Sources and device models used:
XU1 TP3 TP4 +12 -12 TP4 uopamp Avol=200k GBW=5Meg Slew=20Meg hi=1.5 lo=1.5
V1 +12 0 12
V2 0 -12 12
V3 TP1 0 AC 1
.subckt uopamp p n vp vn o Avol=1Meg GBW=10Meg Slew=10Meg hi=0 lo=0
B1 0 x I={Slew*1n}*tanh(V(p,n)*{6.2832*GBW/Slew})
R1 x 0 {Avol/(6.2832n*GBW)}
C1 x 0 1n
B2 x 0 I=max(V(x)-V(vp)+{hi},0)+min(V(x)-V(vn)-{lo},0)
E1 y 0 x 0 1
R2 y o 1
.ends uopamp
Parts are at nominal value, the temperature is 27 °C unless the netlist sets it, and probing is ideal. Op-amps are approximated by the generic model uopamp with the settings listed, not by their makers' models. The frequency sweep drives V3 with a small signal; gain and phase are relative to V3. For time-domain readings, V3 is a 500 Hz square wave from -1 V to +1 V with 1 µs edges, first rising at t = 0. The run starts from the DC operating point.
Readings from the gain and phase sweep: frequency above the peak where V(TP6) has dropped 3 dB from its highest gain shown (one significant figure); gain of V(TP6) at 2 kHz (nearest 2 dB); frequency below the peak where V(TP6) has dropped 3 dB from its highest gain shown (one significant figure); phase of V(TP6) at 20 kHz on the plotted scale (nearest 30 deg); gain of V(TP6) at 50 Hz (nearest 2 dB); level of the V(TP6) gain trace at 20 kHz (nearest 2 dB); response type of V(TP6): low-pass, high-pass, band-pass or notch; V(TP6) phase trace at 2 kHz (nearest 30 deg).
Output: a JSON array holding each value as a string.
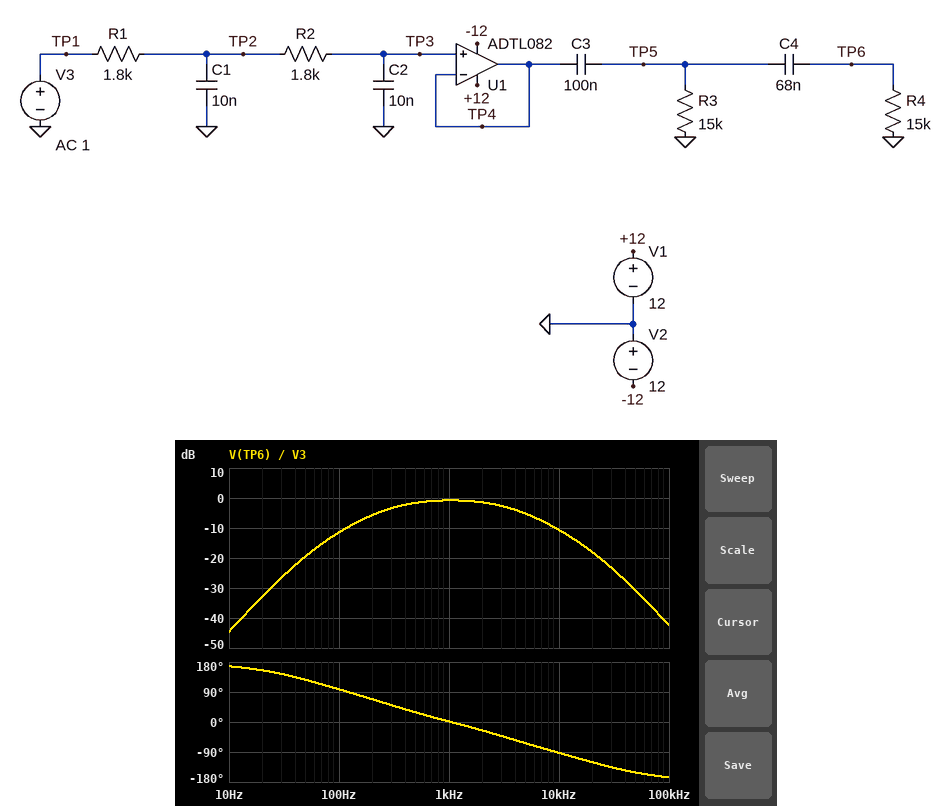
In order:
["4 kHz", "-2 dB", "300 Hz", "-120 deg", "-20 dB", "-18 dB", "band-pass", "-30 deg"]
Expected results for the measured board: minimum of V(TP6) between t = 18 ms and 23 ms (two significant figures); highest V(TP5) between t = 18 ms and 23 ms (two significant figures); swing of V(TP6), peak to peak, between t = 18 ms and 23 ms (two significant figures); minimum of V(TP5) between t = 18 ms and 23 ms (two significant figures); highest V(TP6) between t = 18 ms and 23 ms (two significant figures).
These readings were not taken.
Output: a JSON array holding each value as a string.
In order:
["-1.4 V", "1.2 V", "2.9 V", "-1.2 V", "1.4 V"]
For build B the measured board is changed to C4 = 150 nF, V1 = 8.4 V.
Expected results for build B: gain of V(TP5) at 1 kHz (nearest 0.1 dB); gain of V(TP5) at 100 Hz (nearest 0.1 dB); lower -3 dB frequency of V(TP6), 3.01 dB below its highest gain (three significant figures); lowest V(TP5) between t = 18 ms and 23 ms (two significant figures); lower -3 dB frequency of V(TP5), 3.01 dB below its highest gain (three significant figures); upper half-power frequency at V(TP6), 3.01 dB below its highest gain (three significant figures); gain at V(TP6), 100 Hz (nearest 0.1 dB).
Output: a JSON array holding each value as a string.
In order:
["-0.6 dB", "-7.3 dB", "225 Hz", "-1.3 V", "206 Hz", "3.77 kHz", "-9.1 dB"]
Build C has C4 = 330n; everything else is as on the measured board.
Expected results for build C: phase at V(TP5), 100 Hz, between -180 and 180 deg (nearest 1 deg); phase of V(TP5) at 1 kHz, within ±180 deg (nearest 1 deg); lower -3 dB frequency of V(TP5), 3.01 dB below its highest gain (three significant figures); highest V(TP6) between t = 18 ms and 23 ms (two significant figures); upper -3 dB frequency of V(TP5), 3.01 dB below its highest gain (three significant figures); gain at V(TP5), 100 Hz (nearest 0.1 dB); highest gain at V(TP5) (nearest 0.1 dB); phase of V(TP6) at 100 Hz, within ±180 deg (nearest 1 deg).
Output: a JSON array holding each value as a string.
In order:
["55 deg", "-7 deg", "200 Hz", "1.3 V", "3.72 kHz", "-7.6 dB", "-0.6 dB", "73 deg"]
